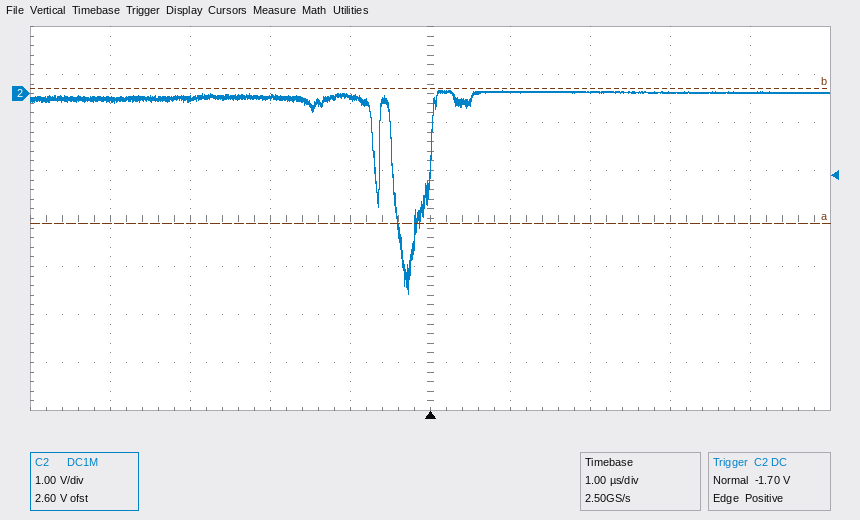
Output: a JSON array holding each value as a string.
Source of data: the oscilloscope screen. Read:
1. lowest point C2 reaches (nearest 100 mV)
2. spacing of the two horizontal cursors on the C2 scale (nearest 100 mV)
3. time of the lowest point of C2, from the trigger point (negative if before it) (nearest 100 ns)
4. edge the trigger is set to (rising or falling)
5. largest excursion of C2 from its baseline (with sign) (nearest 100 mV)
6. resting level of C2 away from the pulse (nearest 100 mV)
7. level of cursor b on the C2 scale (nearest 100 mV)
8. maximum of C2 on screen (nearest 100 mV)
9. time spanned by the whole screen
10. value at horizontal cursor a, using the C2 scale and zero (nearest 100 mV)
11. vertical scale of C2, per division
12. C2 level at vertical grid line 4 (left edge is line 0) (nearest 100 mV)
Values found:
["-4.2 V", "2.8 V", "-300 ns", "rising", "-4.2 V", "0.0 V", "100 mV", "100 mV", "10 µs", "-2.7 V", "1 V", "-100 mV"]
